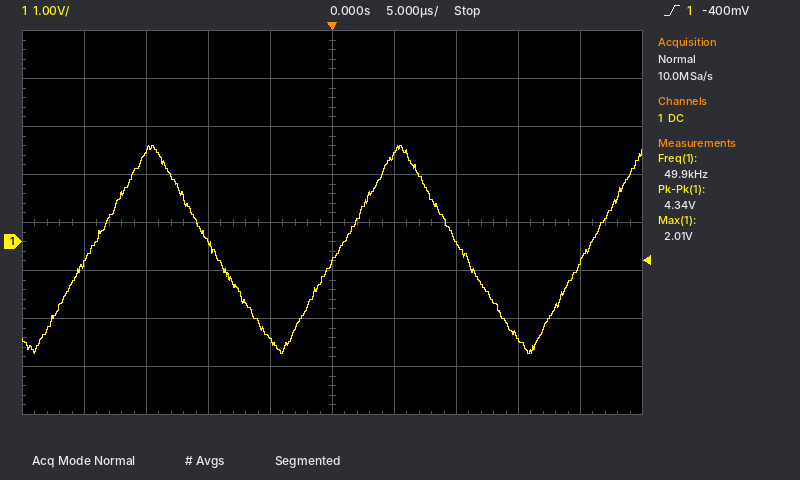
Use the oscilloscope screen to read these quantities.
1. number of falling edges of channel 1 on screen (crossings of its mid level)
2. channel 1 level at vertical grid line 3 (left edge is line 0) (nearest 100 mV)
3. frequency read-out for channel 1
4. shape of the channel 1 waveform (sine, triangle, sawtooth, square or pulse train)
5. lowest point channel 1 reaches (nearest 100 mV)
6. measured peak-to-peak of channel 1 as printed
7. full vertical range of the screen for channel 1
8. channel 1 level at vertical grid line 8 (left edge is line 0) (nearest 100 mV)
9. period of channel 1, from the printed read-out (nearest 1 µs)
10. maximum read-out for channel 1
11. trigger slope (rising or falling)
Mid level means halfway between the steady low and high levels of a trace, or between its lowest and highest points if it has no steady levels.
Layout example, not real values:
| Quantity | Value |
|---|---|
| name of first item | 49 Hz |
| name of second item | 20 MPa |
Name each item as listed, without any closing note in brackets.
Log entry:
| Quantity | Value |
|---|---|
| number of falling edges of channel 1 on screen | 2 |
| channel 1 level at vertical grid line 3 (left edge is line 0) | 0.0 V |
| frequency read-out for channel 1 | 49.9 kHz |
| shape of the channel 1 waveform | triangle |
| lowest point channel 1 reaches | -2.3 V |
| measured peak-to-peak of channel 1 as printed | 4.34 V |
| full vertical range of the screen for channel 1 | 8 V |
| channel 1 level at vertical grid line 8 (left edge is line 0) | -2.0 V |
| period of channel 1, from the printed read-out | 20 µs |
| maximum read-out for channel 1 | 2.01 V |
| trigger slope | rising |
